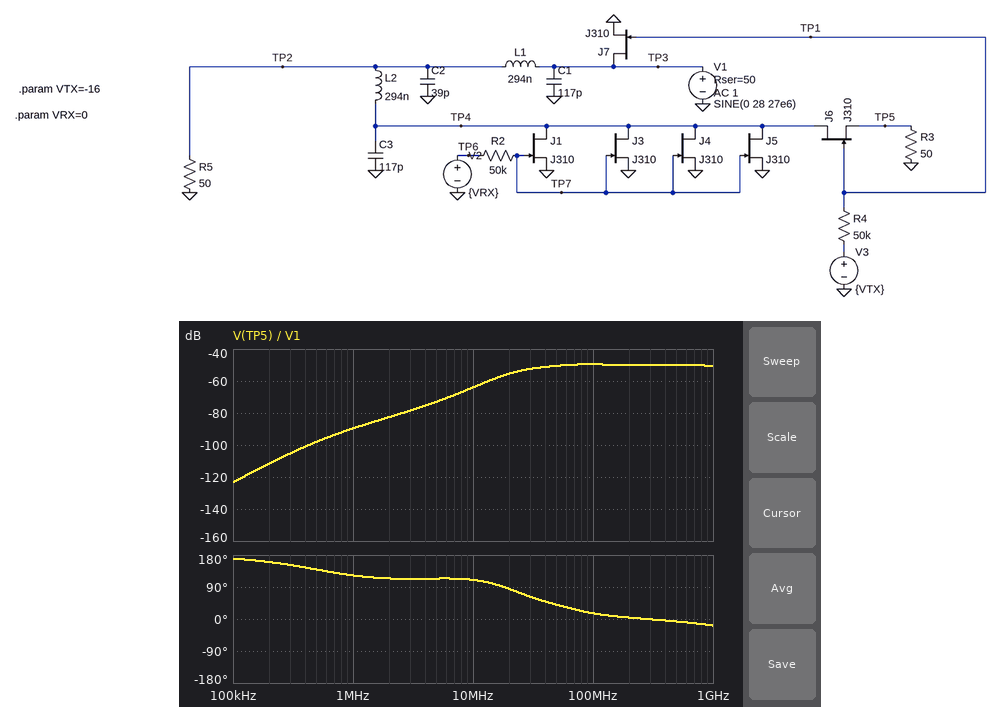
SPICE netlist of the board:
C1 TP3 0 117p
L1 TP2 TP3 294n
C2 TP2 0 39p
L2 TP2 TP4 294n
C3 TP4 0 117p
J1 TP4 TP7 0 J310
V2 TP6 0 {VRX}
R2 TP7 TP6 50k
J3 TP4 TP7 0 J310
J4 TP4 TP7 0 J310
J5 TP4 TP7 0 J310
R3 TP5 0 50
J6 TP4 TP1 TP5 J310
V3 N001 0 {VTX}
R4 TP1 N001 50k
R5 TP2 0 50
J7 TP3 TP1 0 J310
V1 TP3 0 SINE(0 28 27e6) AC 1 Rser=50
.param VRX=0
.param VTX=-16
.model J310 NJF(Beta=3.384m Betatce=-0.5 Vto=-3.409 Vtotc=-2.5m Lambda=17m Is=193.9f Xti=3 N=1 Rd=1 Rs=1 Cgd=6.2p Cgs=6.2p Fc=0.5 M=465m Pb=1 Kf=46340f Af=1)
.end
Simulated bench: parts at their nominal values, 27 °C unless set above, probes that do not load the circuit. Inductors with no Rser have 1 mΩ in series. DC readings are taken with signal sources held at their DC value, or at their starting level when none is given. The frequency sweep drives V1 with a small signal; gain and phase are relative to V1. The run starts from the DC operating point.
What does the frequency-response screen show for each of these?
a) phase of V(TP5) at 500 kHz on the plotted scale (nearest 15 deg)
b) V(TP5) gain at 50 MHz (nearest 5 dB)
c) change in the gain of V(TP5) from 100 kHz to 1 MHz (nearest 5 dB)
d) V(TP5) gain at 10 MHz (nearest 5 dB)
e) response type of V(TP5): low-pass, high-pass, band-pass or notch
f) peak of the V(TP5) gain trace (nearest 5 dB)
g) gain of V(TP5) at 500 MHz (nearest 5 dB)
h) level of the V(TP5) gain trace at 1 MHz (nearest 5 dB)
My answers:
135 deg
-50 dB
35 dB
-65 dB
high-pass
-50 dB
-50 dB
-90 dB
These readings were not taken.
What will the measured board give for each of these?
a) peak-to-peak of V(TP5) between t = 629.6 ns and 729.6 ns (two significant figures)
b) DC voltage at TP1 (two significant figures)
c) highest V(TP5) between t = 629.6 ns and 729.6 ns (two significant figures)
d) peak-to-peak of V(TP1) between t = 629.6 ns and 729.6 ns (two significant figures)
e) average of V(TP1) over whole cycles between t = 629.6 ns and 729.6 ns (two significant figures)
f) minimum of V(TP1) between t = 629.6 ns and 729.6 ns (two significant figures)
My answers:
140 mV
-16 V
64 mV
11 V
-16 V
-22 V
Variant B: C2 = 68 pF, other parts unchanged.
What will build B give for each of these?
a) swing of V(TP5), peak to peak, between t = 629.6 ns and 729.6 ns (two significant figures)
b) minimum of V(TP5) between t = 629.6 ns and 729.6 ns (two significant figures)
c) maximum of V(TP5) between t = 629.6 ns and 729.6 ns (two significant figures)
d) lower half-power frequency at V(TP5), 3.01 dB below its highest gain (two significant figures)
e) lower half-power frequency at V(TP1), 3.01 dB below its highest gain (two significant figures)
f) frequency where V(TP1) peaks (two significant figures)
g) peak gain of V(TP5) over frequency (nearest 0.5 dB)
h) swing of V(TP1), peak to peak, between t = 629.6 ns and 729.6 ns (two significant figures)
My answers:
130 mV
-68 mV
60 mV
34 MHz
8.5 MHz
21 MHz
-49.5 dB
9.9 V
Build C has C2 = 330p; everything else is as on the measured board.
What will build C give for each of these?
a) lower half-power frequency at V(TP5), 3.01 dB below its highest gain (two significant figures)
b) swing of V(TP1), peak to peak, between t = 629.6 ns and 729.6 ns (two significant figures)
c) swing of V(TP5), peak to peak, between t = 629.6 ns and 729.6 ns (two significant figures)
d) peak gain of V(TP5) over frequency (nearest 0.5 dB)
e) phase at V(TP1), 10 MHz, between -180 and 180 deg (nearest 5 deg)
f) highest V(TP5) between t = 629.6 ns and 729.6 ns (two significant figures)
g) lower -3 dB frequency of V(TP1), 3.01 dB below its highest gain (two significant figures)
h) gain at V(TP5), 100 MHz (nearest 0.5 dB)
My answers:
31 MHz
7.9 V
100 mV
-48.5 dB
10 deg
56 mV
28 MHz
-49.5 dB
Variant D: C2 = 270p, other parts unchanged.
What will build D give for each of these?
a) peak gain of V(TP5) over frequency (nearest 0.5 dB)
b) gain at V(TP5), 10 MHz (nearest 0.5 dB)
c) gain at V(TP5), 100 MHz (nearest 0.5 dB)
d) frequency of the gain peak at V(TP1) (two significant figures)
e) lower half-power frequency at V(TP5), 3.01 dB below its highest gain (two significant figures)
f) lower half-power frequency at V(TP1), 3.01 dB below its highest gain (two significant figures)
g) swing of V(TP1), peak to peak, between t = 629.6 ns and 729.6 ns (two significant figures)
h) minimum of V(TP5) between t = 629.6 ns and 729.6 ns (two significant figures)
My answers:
-48.5 dB
-64.5 dB
-49.5 dB
37 MHz
32 MHz
29 MHz
6.6 V
-43 mV
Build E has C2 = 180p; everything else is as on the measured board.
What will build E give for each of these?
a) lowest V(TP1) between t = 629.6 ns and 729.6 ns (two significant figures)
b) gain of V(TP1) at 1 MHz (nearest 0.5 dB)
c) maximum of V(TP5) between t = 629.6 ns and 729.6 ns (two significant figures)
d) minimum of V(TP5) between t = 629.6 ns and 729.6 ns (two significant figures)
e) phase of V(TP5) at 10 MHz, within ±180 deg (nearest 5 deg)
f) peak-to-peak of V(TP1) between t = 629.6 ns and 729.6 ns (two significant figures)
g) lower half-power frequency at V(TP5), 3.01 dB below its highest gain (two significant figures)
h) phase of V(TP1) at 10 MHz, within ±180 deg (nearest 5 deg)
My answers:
-20 V
-23.0 dB
45 mV
-49 mV
105 deg
6.9 V
36 MHz
15 deg
